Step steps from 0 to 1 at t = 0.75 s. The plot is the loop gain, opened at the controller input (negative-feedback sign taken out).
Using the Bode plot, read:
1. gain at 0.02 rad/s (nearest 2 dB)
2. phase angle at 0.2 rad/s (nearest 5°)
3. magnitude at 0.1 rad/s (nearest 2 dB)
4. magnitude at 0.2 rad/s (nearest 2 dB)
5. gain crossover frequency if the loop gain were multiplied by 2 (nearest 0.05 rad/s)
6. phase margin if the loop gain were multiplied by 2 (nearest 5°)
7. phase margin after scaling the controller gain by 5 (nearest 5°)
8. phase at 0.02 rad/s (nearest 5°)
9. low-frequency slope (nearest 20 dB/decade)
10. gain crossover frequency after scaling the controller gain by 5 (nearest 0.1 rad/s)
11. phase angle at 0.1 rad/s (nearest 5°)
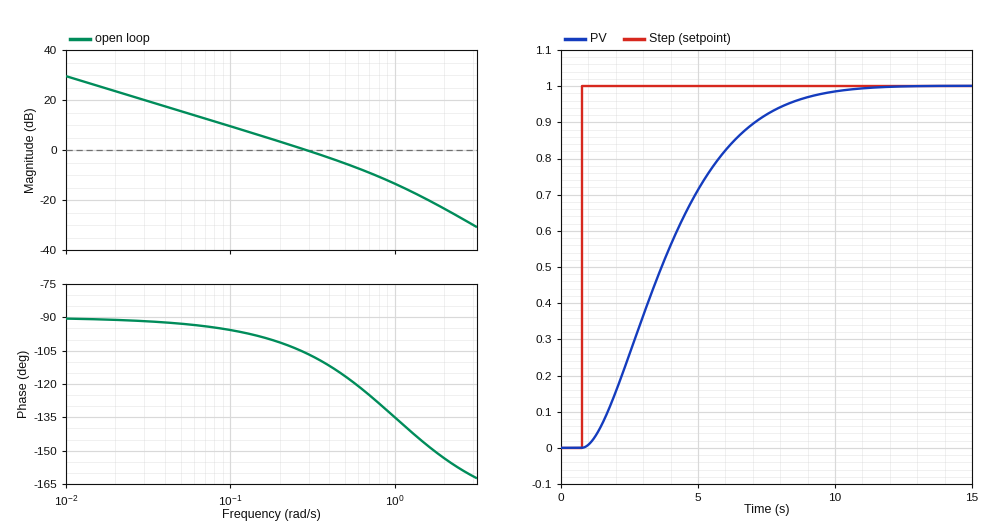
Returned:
24 dB
-100°
10 dB
4 dB
0.55 rad/s
60°
45°
-90°
-20 dB/decade
1.0 rad/s
-95°
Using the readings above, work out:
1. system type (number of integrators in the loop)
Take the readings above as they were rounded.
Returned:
1
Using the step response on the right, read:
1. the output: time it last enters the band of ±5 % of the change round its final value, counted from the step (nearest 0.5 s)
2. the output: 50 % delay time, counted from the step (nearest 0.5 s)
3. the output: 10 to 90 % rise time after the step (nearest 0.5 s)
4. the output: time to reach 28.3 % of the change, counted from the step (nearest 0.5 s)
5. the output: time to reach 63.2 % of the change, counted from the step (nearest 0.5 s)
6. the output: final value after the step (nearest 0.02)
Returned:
7.5 s
3.0 s
5.5 s
2.0 s
3.5 s
1.00
